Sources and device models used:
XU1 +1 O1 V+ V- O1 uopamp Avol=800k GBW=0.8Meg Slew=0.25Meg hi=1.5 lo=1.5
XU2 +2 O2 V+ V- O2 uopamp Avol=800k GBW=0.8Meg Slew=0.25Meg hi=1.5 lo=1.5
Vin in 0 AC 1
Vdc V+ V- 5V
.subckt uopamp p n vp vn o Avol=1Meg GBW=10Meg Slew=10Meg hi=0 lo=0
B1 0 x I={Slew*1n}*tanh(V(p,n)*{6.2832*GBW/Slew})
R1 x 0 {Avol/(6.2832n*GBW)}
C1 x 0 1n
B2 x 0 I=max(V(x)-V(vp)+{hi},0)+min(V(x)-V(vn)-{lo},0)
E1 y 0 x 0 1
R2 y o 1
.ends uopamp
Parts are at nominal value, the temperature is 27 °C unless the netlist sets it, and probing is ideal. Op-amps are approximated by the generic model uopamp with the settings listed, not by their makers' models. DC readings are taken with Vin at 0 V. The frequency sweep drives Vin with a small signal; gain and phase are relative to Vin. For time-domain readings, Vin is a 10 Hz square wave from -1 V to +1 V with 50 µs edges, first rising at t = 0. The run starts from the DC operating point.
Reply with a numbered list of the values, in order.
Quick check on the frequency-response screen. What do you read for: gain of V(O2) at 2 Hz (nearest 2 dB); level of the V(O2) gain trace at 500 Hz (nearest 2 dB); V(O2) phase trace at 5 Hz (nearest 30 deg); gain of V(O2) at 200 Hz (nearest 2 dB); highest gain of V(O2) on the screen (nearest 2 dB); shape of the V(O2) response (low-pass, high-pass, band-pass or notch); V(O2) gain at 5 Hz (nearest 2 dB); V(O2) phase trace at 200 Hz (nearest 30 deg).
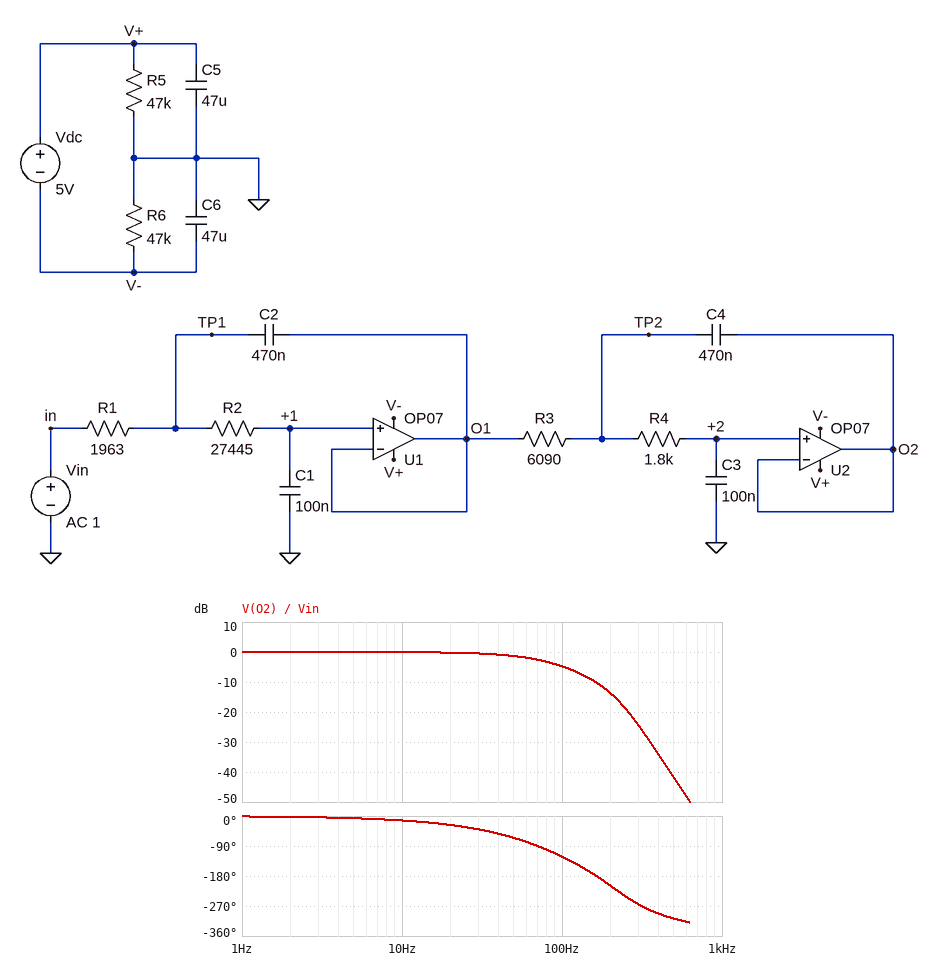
1. 0 dB
2. -42 dB
3. 0 deg
4. -14 dB
5. 0 dB
6. low-pass
7. 0 dB
8. -210 deg
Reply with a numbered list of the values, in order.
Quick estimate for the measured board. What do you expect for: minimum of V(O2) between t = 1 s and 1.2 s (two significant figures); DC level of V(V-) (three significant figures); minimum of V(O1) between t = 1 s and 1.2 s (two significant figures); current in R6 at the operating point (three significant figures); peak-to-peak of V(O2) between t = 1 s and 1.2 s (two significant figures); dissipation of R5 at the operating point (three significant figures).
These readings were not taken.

1. -1.0 V
2. -2.50 V
3. -1.0 V
4. 53.2 µA
5. 2.0 V
6. 133 µW
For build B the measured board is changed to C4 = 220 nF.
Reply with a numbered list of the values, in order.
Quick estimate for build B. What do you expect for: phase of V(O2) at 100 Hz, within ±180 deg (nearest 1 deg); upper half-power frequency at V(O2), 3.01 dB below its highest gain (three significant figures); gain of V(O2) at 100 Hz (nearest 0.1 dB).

1. -119 deg
2. 70.3 Hz
3. -5.6 dB
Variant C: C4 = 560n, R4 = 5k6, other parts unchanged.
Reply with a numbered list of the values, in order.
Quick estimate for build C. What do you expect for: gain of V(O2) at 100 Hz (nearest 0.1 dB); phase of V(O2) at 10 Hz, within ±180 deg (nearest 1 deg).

1. -3.1 dB
2. -15 deg
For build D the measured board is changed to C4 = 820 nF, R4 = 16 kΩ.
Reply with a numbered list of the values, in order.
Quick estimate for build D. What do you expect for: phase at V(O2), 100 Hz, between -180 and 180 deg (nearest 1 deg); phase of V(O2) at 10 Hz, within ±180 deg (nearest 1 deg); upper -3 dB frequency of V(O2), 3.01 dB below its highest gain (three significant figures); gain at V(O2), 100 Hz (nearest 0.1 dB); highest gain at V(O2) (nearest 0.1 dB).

1. 123 deg
2. -19 deg
3. 62.5 Hz
4. -13.5 dB
5. 1.6 dB
